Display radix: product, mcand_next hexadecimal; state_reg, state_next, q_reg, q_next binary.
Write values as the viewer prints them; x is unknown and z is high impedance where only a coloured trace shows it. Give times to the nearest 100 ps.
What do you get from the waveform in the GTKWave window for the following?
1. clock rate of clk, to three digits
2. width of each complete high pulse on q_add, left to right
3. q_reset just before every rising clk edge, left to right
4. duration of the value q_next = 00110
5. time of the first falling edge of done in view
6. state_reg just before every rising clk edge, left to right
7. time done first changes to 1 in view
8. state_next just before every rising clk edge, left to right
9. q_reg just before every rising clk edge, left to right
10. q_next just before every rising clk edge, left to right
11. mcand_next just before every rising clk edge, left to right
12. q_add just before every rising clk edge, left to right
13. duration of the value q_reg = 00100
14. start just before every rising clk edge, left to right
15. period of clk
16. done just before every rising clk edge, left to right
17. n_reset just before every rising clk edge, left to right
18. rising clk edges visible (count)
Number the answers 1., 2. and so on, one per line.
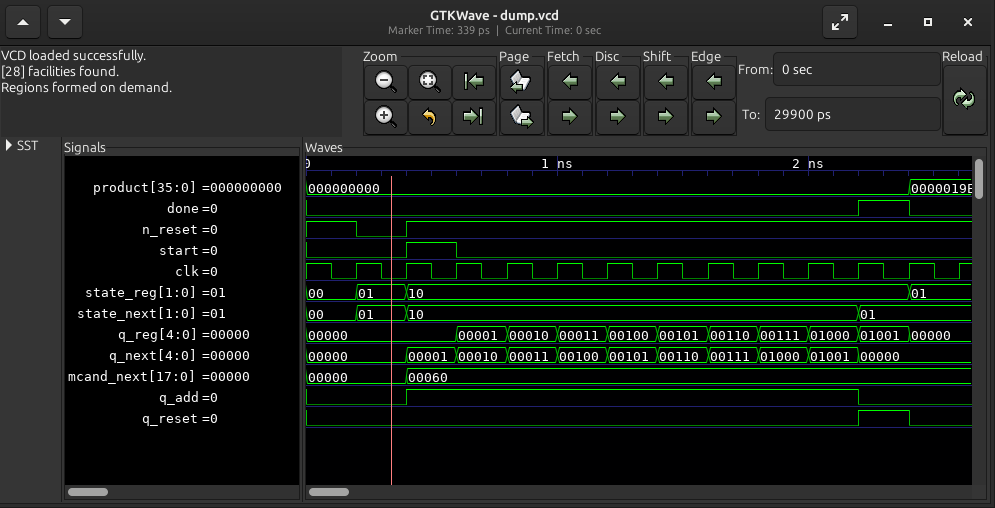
1. 5.00 GHz
2. 1800 ps
3. 0 0 0 0 0 0 0 0 0 0 0 1 0
4. 200 ps
5. 2400 ps
6. 00, 01, 10, 10, 10, 10, 10, 10, 10, 10, 10, 10, 01
7. 2200 ps
8. 00, 01, 10, 10, 10, 10, 10, 10, 10, 10, 10, 01, 01
9. 00000, 00000, 00000, 00001, 00010, 00011, 00100, 00101, 00110, 00111, 01000, 01001, 00000
10. 00000, 00000, 00001, 00010, 00011, 00100, 00101, 00110, 00111, 01000, 01001, 00000, 00000
11. 00000, 00000, 00060, 00060, 00060, 00060, 00060, 00060, 00060, 00060, 00060, 00060, 00060
12. 0 0 1 1 1 1 1 1 1 1 1 0 0
13. 200 ps
14. 0 0 1 0 0 0 0 0 0 0 0 0 0
15. 200 ps
16. 0 0 0 0 0 0 0 0 0 0 0 1 0
17. 1 0 1 1 1 1 1 1 1 1 1 1 1
18. 13
